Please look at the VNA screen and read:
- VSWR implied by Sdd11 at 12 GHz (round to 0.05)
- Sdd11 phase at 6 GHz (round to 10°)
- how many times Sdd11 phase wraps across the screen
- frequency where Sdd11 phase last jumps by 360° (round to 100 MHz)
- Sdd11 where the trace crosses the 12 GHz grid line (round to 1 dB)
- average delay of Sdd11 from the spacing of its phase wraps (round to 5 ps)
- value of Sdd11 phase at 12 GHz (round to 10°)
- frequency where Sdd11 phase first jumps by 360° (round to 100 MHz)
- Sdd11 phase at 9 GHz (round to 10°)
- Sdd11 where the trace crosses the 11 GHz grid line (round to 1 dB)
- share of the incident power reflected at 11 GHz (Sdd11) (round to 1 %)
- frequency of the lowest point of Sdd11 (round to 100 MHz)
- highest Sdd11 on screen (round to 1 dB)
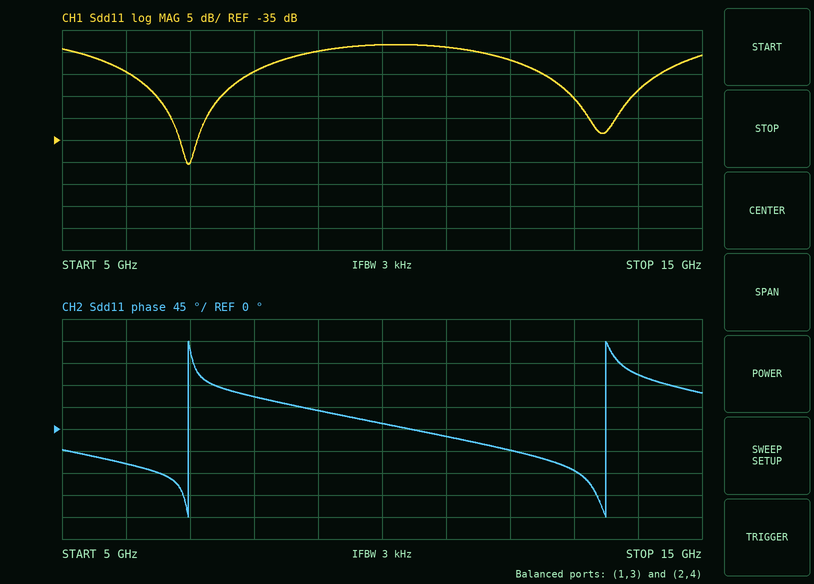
1.35
-70°
2
13.5 GHz
-17 dB
155 ps
-40°
7.0 GHz
40°
-14 dB
4 %
7.0 GHz
-13 dB
